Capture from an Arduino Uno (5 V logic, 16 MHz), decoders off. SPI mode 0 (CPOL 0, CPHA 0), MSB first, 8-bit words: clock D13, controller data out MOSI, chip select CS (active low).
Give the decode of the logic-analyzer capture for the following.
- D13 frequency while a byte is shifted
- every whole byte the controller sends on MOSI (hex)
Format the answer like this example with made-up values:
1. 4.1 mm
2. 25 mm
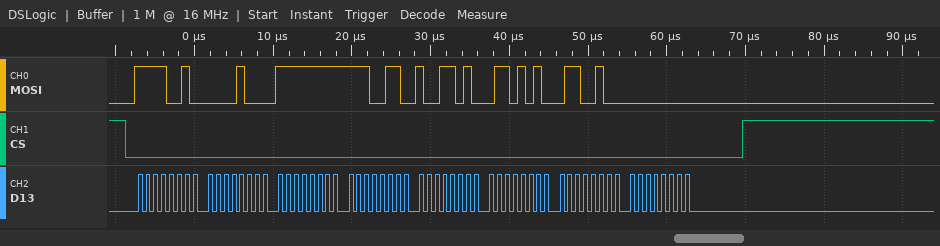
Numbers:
1. 1 MHz
2. F2 08 FF E6 9A 6A 64 00
